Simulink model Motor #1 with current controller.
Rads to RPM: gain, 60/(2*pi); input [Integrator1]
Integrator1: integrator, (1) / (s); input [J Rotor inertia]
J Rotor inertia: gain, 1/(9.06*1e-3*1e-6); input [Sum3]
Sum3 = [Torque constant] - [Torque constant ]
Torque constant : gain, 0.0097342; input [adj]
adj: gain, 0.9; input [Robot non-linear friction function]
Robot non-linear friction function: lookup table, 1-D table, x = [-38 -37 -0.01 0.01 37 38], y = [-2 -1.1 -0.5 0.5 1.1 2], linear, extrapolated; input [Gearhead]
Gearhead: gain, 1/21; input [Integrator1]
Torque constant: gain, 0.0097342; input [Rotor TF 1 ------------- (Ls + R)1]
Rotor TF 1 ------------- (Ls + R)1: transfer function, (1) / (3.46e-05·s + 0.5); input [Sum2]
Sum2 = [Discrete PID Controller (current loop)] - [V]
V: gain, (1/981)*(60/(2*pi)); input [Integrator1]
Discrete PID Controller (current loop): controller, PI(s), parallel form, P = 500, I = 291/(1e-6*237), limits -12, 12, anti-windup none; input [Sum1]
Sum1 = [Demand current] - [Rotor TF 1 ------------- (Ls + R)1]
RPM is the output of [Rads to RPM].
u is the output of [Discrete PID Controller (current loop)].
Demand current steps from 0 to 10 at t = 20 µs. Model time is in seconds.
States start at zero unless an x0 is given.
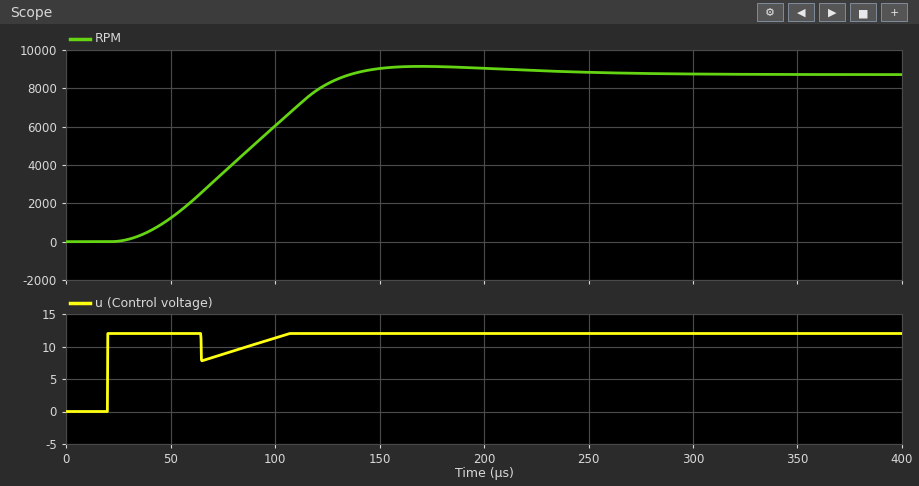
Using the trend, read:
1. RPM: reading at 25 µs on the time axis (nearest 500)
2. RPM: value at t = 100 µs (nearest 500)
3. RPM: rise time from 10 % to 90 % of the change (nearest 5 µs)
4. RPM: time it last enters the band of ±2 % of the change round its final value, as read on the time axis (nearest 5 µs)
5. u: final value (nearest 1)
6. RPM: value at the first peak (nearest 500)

0
6000
75 µs
235 µs
12
9000
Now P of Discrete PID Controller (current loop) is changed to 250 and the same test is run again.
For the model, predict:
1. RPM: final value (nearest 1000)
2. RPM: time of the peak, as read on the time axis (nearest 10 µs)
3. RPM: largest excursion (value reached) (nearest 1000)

9000
170 µs
9000
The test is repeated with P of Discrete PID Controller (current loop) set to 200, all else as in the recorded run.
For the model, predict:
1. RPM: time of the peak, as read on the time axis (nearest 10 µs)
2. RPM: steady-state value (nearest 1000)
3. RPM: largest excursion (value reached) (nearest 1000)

170 µs
9000
9000
